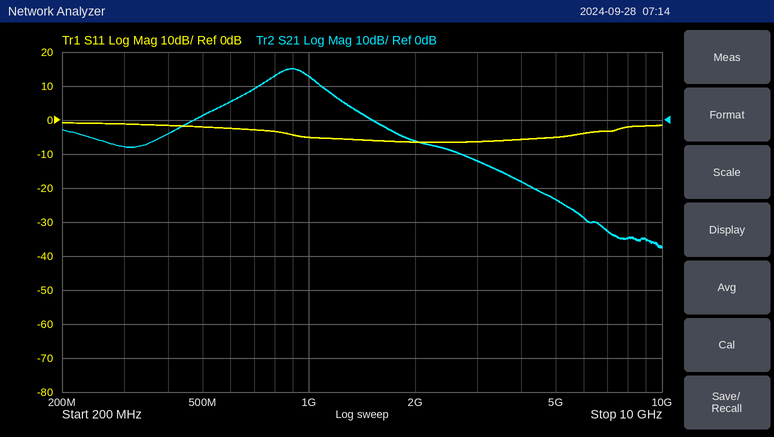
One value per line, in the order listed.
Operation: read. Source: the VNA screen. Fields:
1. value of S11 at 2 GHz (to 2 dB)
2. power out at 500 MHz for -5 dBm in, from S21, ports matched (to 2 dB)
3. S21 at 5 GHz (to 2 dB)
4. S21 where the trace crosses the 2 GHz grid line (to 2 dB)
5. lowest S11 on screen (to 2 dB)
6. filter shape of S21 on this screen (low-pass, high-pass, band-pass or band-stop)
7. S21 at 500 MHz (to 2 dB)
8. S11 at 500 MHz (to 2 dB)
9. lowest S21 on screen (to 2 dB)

-6 dB
-4 dBm
-24 dB
-6 dB
-6 dB
band-pass
2 dB
-2 dB
-38 dB
